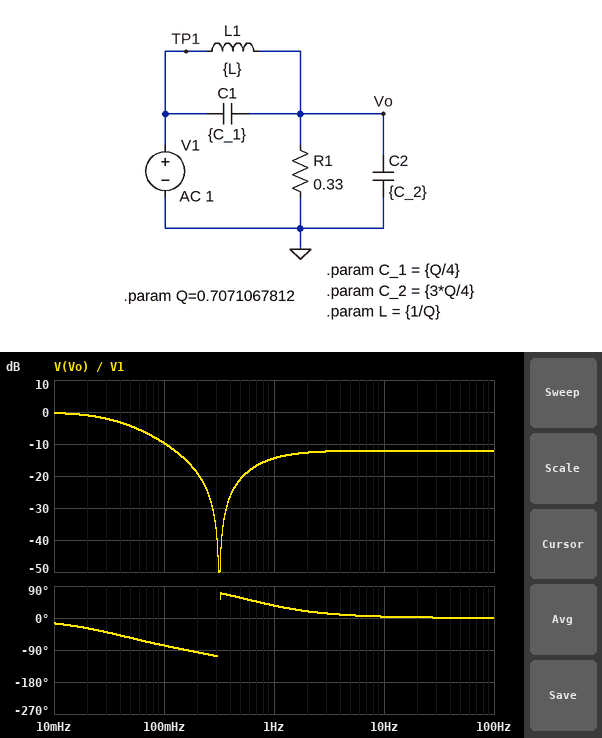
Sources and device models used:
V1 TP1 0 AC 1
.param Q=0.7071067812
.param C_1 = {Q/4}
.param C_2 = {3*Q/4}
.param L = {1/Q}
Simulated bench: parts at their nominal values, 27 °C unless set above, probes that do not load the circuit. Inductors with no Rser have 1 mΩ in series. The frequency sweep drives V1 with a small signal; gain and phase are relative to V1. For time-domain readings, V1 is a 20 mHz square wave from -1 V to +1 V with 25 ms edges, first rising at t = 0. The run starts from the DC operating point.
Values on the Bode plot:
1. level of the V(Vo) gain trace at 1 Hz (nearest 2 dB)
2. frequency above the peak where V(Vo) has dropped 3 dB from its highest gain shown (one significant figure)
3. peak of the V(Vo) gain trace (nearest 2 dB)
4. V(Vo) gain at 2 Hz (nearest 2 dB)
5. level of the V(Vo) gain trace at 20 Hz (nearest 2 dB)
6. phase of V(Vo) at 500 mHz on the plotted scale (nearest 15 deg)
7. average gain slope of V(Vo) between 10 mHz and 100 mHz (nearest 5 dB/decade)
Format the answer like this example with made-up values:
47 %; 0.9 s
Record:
-14 dB; 40 mHz; 0 dB; -12 dB; -12 dB; 60 deg; -10 dB/decade
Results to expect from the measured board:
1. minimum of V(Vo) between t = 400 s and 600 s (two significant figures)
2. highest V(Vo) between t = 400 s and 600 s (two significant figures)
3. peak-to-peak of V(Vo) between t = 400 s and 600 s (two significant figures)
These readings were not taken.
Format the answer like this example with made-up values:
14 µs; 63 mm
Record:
-990 mV; 990 mV; 2.0 V
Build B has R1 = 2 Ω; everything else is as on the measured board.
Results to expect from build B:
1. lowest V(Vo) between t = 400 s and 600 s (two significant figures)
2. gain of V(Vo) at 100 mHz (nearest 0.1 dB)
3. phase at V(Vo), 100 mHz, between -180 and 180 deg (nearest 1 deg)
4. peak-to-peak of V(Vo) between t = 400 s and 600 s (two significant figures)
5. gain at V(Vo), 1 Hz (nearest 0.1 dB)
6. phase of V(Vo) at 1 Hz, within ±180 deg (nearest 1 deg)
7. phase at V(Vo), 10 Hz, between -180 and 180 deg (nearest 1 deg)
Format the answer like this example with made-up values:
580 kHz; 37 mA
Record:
-1.5 V; 1.6 dB; -36 deg; 2.9 V; -12.8 dB; 7 deg; 1 deg
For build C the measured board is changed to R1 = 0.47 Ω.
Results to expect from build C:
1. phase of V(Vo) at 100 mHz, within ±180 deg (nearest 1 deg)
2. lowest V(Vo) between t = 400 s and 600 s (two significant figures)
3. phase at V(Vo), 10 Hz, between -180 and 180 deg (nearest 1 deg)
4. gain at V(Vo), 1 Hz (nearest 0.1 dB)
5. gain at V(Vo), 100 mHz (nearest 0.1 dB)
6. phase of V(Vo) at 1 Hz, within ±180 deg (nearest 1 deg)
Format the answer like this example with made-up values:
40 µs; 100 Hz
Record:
-72 deg; -1.0 V; 3 deg; -13.7 dB; -6.9 dB; 26 deg
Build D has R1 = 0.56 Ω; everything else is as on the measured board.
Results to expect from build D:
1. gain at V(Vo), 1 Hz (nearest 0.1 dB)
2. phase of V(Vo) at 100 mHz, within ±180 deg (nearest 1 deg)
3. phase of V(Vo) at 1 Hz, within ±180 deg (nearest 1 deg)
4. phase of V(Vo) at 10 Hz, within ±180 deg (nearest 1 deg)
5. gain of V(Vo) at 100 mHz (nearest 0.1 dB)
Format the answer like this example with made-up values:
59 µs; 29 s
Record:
-13.4 dB; -69 deg; 22 deg; 2 deg; -5.5 dB
